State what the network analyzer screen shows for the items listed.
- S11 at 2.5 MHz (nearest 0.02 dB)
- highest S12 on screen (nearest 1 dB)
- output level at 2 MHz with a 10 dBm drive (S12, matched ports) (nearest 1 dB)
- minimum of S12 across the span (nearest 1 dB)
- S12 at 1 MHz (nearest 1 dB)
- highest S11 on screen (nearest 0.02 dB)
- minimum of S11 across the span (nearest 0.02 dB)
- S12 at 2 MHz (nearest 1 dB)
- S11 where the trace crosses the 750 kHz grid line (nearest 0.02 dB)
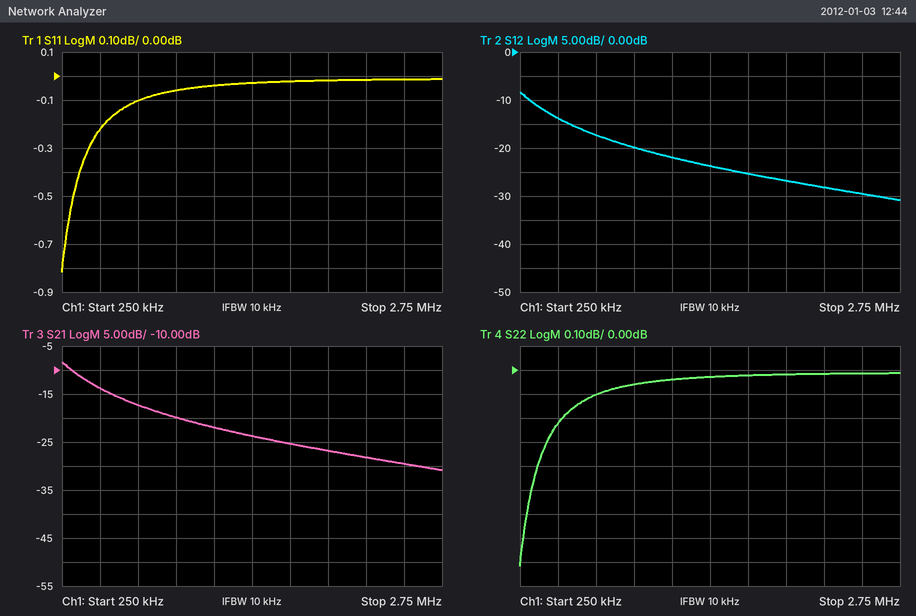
-0.02 dB
-8 dB
-17 dBm
-31 dB
-20 dB
-0.02 dB
-0.82 dB
-27 dB
-0.10 dB
